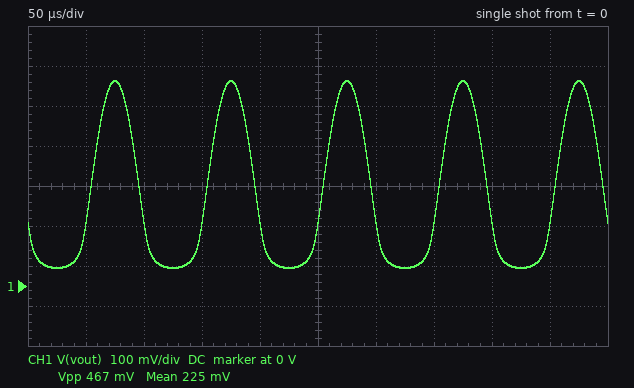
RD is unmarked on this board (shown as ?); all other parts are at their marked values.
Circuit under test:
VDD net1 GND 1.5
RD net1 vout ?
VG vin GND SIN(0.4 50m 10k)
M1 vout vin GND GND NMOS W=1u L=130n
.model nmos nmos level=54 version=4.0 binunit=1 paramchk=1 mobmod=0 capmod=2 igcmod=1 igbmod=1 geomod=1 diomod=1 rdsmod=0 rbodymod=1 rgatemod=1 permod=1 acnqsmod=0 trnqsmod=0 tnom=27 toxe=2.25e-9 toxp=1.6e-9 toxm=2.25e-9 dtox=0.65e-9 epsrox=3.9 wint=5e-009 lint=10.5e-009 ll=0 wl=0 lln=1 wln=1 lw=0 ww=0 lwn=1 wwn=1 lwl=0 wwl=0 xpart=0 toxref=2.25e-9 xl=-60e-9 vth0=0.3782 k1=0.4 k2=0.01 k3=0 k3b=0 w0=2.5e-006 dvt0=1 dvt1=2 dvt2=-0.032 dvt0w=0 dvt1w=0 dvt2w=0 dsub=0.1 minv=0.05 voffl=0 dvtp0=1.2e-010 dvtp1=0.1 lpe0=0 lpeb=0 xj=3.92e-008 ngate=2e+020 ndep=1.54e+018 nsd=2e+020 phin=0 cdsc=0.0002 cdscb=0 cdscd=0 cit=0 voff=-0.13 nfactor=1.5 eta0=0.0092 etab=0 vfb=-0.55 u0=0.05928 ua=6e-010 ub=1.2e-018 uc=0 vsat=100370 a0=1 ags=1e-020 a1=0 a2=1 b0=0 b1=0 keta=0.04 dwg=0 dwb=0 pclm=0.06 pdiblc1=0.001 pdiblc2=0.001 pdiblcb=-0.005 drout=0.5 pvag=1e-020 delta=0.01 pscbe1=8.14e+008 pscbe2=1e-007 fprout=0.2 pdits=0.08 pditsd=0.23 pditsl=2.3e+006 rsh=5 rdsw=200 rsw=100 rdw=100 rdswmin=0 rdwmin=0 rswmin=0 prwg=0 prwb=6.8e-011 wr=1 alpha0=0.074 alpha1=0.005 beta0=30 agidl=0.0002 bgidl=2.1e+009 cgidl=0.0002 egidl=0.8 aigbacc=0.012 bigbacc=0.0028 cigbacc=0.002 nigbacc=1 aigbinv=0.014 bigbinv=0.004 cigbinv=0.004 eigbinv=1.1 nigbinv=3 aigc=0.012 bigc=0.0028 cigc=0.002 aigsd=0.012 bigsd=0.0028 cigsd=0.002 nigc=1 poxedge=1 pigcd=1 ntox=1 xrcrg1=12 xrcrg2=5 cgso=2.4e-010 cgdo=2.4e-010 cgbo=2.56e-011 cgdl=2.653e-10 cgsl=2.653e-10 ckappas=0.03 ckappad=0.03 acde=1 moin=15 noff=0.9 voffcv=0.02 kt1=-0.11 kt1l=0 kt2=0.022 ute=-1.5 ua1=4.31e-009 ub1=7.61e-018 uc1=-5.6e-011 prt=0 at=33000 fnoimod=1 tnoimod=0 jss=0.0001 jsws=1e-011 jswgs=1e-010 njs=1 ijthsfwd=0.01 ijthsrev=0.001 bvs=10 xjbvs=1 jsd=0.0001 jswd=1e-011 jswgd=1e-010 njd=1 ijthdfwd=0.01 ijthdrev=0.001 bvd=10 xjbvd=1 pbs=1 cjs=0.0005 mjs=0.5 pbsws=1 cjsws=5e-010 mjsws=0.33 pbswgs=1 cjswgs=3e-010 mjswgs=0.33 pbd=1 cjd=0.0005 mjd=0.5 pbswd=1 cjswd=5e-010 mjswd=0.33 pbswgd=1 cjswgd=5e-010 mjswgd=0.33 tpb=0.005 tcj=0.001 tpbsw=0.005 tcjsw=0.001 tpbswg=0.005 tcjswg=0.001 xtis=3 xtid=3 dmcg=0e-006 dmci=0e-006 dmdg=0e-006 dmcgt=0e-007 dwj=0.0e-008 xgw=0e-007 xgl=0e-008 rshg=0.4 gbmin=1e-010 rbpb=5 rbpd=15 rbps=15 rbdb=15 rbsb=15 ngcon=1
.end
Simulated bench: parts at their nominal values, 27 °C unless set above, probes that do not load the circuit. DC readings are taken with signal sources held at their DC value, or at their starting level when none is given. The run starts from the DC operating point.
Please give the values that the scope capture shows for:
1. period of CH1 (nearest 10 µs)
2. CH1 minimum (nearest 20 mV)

100 µs
40 mV
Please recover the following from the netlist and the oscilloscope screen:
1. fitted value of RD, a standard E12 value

47 kΩ
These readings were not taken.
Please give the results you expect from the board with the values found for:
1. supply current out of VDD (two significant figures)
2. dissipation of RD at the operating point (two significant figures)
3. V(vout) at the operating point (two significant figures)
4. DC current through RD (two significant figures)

29 µA
38 µW
160 mV
29 µA
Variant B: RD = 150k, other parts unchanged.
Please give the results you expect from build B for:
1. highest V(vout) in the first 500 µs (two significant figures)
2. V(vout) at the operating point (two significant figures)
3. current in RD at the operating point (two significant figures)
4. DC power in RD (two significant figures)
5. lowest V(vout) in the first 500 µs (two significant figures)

58 mV
20 mV
9.9 µA
15 µW
12 mV
